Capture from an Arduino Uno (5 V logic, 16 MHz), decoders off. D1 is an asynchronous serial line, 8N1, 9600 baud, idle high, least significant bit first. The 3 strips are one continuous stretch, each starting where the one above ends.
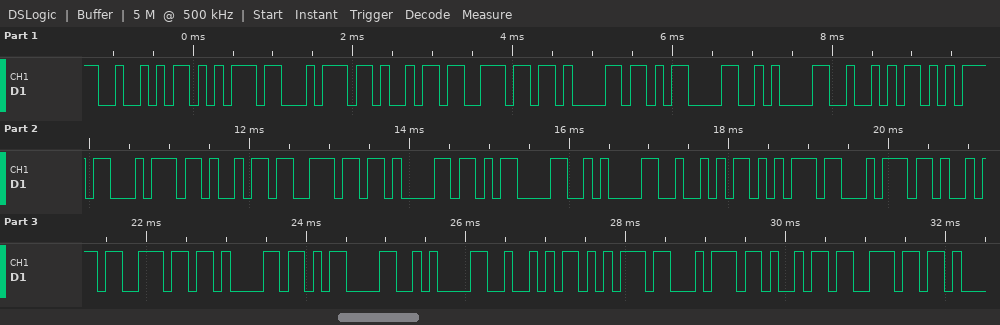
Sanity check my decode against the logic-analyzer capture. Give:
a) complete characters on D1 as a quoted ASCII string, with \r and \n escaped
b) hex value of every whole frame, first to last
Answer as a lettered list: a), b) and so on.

a) "Rutina\r\nRutina\r\nRutina\r\nRutin"
b) 0x52 0x75 0x74 0x69 0x6E 0x61 0x0D 0x0A 0x52 0x75 0x74 0x69 0x6E 0x61 0x0D 0x0A 0x52 0x75 0x74 0x69 0x6E 0x61 0x0D 0x0A 0x52 0x75 0x74 0x69 0x6E
